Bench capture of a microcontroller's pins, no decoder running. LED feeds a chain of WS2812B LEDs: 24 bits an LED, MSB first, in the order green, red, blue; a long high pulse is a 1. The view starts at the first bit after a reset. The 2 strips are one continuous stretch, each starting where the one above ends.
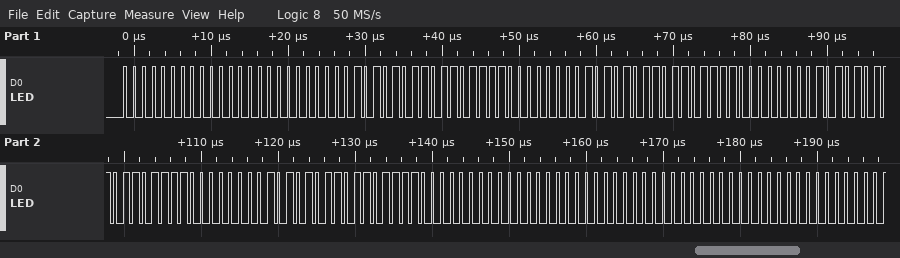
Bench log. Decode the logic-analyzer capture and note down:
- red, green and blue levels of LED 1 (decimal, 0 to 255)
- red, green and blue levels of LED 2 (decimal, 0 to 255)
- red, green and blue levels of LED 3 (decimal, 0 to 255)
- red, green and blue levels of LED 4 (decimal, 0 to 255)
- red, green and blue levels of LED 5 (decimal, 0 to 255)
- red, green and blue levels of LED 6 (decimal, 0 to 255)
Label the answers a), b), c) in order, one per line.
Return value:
a) 0, 0, 0
b) 111, 171, 0
c) 111, 171, 0
d) 111, 171, 0
e) 111, 171, 0
f) 0, 0, 0
